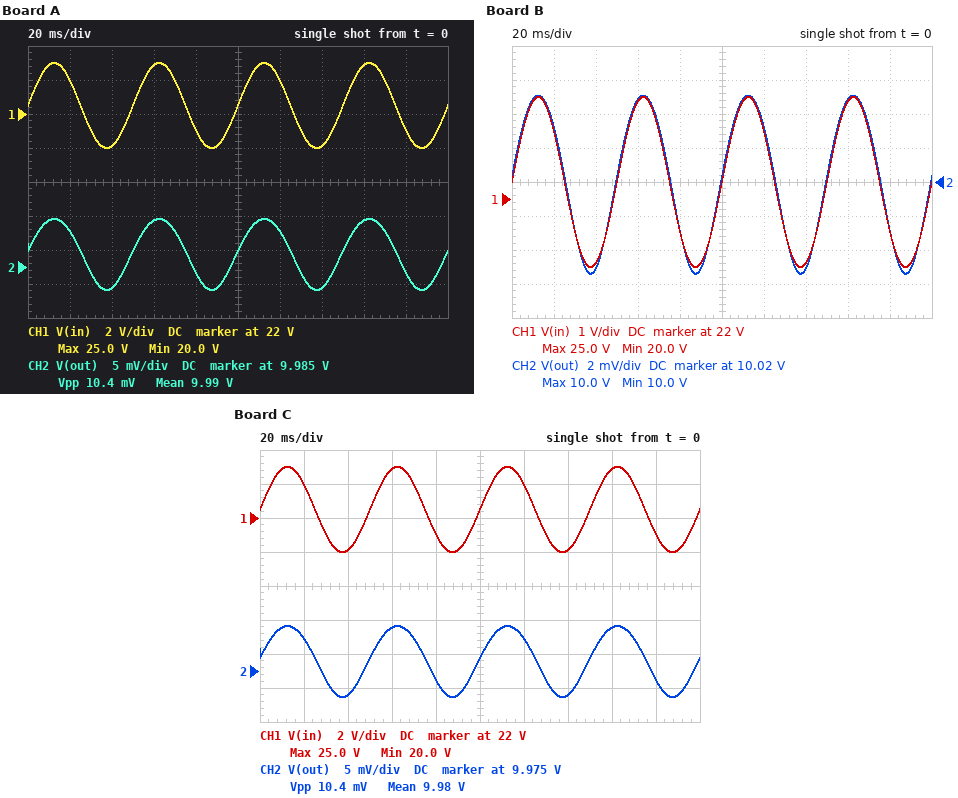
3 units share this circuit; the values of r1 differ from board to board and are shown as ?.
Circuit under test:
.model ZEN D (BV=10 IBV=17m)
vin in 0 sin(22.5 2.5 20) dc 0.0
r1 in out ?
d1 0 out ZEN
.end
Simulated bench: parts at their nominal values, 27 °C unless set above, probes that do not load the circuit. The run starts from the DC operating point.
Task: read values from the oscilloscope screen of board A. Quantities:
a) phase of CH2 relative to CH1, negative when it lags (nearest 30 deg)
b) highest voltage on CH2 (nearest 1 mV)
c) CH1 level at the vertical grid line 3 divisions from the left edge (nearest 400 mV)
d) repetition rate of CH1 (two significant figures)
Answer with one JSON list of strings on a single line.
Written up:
["0 deg", "9.992 V", "24.8 V", "20 Hz"]
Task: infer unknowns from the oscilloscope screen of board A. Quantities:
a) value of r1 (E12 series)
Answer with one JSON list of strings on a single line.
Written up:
["1.2 kΩ"]
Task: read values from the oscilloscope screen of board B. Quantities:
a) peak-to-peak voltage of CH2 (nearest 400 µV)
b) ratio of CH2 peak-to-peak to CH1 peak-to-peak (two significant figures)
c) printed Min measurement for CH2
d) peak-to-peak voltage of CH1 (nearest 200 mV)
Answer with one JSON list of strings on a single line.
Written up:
["10.4 mV", "0.0021", "10.0 V", "5.0 V"]
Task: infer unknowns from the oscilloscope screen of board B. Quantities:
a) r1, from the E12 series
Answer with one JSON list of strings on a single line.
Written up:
["390 Ω"]
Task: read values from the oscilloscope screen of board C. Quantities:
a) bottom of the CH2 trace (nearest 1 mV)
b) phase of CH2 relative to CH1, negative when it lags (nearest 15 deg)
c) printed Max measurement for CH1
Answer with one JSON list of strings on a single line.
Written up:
["9.971 V", "0 deg", "25.0 V"]
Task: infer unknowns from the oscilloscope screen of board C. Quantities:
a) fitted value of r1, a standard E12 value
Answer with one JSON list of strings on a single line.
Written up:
["1.8 kΩ"]
